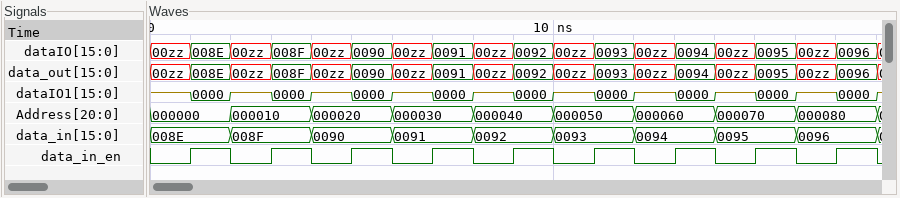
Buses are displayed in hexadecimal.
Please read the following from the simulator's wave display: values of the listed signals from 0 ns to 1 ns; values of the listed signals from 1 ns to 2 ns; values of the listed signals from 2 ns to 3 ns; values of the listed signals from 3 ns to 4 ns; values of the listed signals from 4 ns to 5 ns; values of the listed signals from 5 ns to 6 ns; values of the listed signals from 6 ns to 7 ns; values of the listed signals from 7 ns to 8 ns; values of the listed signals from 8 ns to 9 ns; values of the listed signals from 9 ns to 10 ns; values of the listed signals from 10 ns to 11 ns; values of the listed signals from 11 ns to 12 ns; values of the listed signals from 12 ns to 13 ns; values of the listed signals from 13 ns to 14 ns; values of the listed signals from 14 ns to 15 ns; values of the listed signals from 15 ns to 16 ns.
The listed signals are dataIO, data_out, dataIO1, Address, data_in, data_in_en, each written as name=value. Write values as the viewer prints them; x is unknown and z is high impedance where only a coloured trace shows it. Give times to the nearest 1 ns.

dataIO=00zz, data_out=00zz, dataIO1=z, Address=000000, data_in=008E, data_in_en=0
dataIO=008E, data_out=008E, dataIO1=0000, Address=000000, data_in=008E, data_in_en=1
dataIO=00zz, data_out=00zz, dataIO1=z, Address=000010, data_in=008F, data_in_en=0
dataIO=008F, data_out=008F, dataIO1=0000, Address=000010, data_in=008F, data_in_en=1
dataIO=00zz, data_out=00zz, dataIO1=z, Address=000020, data_in=0090, data_in_en=0
dataIO=0090, data_out=0090, dataIO1=0000, Address=000020, data_in=0090, data_in_en=1
dataIO=00zz, data_out=00zz, dataIO1=z, Address=000030, data_in=0091, data_in_en=0
dataIO=0091, data_out=0091, dataIO1=0000, Address=000030, data_in=0091, data_in_en=1
dataIO=00zz, data_out=00zz, dataIO1=z, Address=000040, data_in=0092, data_in_en=0
dataIO=0092, data_out=0092, dataIO1=0000, Address=000040, data_in=0092, data_in_en=1
dataIO=00zz, data_out=00zz, dataIO1=z, Address=000050, data_in=0093, data_in_en=0
dataIO=0093, data_out=0093, dataIO1=0000, Address=000050, data_in=0093, data_in_en=1
dataIO=00zz, data_out=00zz, dataIO1=z, Address=000060, data_in=0094, data_in_en=0
dataIO=0094, data_out=0094, dataIO1=0000, Address=000060, data_in=0094, data_in_en=1
dataIO=00zz, data_out=00zz, dataIO1=z, Address=000070, data_in=0095, data_in_en=0
dataIO=0095, data_out=0095, dataIO1=0000, Address=000070, data_in=0095, data_in_en=1
